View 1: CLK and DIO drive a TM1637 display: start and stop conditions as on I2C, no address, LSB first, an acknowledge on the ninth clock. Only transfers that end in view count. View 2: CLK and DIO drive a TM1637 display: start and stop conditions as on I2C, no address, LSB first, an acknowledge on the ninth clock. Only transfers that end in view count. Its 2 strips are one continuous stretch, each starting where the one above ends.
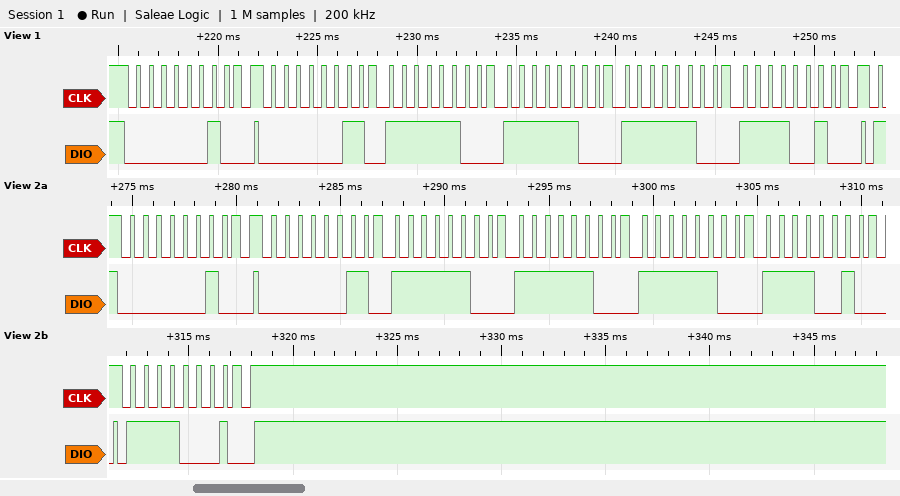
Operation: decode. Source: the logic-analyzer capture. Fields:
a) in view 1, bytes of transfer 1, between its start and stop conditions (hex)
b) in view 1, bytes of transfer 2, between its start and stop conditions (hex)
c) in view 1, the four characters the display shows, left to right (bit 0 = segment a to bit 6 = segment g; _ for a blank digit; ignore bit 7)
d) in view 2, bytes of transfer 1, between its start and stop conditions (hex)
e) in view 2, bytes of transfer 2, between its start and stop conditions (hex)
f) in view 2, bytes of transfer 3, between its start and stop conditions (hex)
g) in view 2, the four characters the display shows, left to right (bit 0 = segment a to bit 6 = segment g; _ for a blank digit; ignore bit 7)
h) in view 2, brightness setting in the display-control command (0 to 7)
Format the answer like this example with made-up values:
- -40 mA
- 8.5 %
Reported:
- 40
- C0 3F 3F 3F 4F
- 0003
- 40
- C0 3F 3F 3F 4F
- 8F
- 0003
- 7
